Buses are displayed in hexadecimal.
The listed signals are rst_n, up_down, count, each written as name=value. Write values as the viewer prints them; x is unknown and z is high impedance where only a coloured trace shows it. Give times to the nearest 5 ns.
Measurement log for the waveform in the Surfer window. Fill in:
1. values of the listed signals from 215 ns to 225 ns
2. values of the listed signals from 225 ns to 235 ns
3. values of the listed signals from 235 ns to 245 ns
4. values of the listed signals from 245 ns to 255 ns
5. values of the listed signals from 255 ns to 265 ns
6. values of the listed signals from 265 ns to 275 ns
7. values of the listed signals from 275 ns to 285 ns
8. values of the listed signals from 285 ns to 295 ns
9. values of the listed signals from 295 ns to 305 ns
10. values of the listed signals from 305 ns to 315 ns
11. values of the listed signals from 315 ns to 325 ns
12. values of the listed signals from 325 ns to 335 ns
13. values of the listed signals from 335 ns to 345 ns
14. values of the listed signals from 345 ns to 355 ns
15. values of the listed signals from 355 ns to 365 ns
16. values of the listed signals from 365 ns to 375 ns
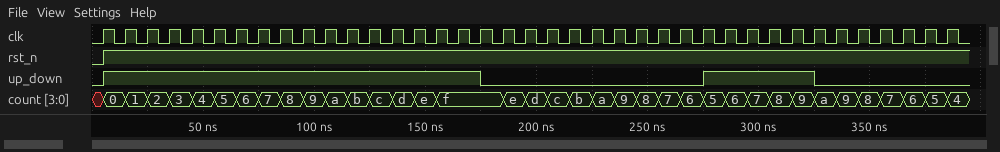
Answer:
rst_n=1, up_down=0, count=b
rst_n=1, up_down=0, count=a
rst_n=1, up_down=0, count=9
rst_n=1, up_down=0, count=8
rst_n=1, up_down=0, count=7
rst_n=1, up_down=0, count=6
rst_n=1, up_down=1, count=5
rst_n=1, up_down=1, count=6
rst_n=1, up_down=1, count=7
rst_n=1, up_down=1, count=8
rst_n=1, up_down=1, count=9
rst_n=1, up_down=0, count=a
rst_n=1, up_down=0, count=9
rst_n=1, up_down=0, count=8
rst_n=1, up_down=0, count=7
rst_n=1, up_down=0, count=6
